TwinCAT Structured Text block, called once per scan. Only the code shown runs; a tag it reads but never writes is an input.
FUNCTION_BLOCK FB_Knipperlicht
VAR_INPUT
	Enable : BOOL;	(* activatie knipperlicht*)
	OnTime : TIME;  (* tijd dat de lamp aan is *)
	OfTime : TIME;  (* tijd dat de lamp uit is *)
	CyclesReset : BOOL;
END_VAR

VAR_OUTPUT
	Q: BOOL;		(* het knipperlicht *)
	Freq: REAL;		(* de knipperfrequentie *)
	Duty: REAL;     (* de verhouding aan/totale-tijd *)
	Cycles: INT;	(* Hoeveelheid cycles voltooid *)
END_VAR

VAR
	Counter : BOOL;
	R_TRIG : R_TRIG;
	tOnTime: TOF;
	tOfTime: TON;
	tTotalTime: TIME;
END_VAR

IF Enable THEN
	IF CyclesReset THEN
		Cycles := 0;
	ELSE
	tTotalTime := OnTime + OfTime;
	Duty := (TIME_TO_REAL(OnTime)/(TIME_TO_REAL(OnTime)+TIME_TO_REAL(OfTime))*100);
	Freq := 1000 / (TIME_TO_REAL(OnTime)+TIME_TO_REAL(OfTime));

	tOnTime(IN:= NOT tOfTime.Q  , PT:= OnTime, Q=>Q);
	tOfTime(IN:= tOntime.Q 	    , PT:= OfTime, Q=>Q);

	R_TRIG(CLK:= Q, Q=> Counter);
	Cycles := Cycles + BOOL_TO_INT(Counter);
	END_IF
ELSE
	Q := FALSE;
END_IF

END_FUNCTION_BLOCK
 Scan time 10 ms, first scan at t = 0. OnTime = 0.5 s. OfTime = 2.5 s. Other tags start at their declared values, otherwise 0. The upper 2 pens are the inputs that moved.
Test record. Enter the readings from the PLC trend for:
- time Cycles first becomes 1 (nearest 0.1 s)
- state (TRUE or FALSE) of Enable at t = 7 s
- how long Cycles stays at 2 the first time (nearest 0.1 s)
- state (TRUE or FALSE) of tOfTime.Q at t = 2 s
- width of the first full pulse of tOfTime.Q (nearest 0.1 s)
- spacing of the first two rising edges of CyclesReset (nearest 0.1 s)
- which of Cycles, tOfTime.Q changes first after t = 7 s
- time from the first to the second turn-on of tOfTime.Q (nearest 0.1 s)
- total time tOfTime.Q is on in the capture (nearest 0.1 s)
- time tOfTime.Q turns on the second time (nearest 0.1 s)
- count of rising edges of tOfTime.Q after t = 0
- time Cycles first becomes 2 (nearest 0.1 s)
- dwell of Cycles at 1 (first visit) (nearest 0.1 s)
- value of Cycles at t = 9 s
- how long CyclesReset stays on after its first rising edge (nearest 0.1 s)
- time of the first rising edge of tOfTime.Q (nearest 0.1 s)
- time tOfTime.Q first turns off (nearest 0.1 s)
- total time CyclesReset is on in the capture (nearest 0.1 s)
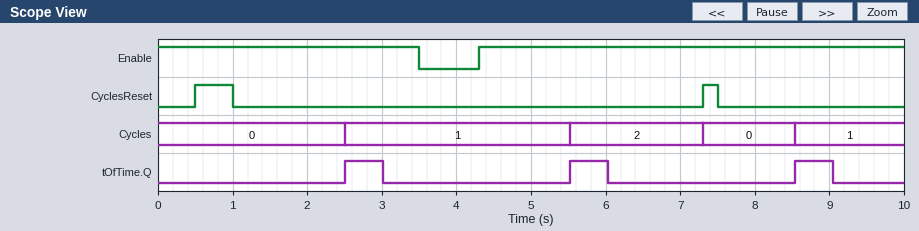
2.5 s
TRUE
1.8 s
FALSE
0.5 s
6.8 s
Cycles
3.0 s
1.5 s
5.5 s
3
5.5 s
3.0 s
1
0.5 s
2.5 s
3.0 s
0.7 s
